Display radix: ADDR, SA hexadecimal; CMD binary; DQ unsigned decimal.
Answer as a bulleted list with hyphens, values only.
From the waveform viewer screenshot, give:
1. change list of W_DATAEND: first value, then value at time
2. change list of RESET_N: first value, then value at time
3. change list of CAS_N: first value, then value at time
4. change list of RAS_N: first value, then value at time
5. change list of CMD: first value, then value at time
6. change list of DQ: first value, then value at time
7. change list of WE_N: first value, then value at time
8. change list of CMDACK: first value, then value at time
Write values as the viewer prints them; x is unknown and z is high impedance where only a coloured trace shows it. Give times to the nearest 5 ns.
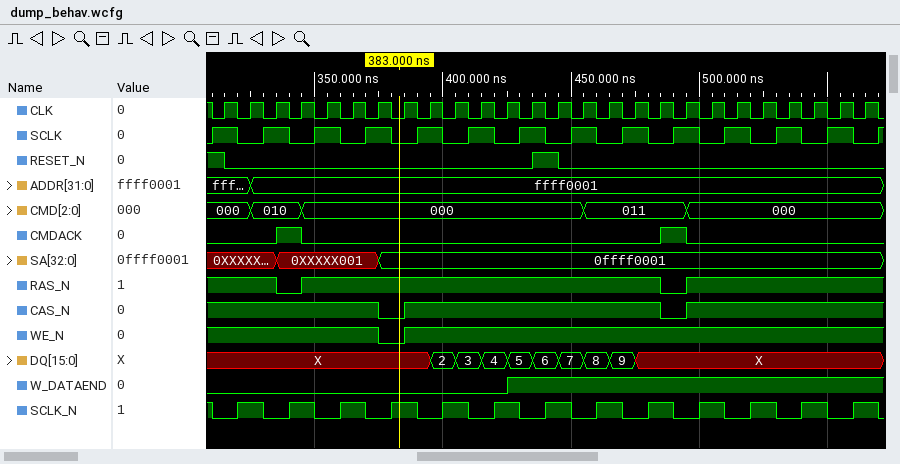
- 0, 1 at 425 ns
- 1, 0 at 315 ns, 1 at 435 ns, 0 at 445 ns
- 1, 0 at 375 ns, 1 at 385 ns, 0 at 485 ns, 1 at 495 ns
- 1, 0 at 335 ns, 1 at 345 ns, 0 at 485 ns, 1 at 495 ns
- 000, 010 at 325 ns, 000 at 345 ns, 011 at 455 ns, 000 at 495 ns
- X, 2 at 395 ns, 3 at 405 ns, 4 at 415 ns, 5 at 425 ns, 6 at 435 ns, 7 at 445 ns, 8 at 455 ns, 9 at 465 ns, X at 475 ns
- 1, 0 at 375 ns, 1 at 385 ns
- 0, 1 at 335 ns, 0 at 345 ns, 1 at 485 ns, 0 at 495 ns
